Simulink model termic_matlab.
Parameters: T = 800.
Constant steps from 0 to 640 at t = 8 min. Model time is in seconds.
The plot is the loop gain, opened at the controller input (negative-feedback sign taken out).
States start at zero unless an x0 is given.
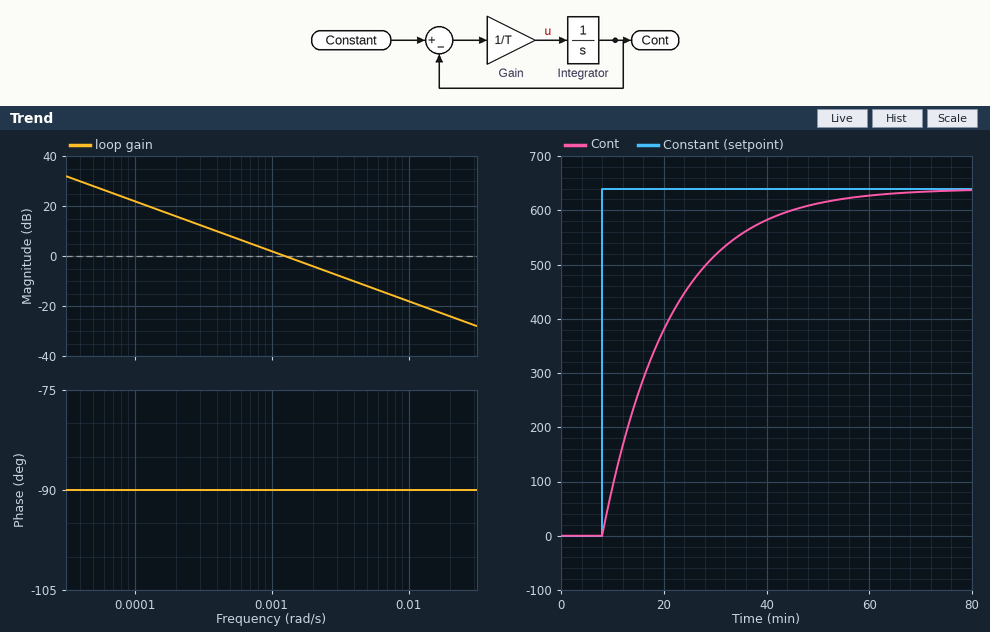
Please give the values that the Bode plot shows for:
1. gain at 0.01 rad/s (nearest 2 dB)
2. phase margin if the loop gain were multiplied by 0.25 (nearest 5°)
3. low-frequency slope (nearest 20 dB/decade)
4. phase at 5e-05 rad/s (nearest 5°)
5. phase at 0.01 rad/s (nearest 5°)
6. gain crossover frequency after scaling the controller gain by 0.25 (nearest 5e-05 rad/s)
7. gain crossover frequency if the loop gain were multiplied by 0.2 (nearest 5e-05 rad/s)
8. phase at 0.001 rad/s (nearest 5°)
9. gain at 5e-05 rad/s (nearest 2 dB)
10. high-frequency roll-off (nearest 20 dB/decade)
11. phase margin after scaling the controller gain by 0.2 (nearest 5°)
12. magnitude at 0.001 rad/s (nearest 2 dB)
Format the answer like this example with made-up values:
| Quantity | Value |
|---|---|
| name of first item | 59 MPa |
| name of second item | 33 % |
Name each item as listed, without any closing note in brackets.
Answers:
| Quantity | Value |
|---|---|
| gain at 0.01 rad/s | -18 dB |
| phase margin if the loop gain were multiplied by 0.25 | 90° |
| low-frequency slope | -20 dB/decade |
| phase at 5e-05 rad/s | -90° |
| phase at 0.01 rad/s | -90° |
| gain crossover frequency after scaling the controller gain by 0.25 | 0.00030 rad/s |
| gain crossover frequency if the loop gain were multiplied by 0.2 | 0.00025 rad/s |
| phase at 0.001 rad/s | -90° |
| gain at 5e-05 rad/s | 28 dB |
| high-frequency roll-off | -20 dB/decade |
| phase margin after scaling the controller gain by 0.2 | 90° |
| magnitude at 0.001 rad/s | 2 dB |
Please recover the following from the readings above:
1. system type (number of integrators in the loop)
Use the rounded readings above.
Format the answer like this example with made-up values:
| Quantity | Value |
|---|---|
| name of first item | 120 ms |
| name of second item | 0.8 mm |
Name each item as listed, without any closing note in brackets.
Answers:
| Quantity | Value |
|---|---|
| system type | 1 |
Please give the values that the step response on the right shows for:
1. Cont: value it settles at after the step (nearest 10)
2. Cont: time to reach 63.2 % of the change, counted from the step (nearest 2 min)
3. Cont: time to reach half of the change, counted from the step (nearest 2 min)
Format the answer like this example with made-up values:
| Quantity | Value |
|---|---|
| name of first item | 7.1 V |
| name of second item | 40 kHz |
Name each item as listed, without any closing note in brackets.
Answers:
| Quantity | Value |
|---|---|
| Cont: value it settles at after the step | 640 |
| Cont: time to reach 63.2 % of the change, counted from the step | 14 min |
| Cont: time to reach half of the change, counted from the step | 10 min |
